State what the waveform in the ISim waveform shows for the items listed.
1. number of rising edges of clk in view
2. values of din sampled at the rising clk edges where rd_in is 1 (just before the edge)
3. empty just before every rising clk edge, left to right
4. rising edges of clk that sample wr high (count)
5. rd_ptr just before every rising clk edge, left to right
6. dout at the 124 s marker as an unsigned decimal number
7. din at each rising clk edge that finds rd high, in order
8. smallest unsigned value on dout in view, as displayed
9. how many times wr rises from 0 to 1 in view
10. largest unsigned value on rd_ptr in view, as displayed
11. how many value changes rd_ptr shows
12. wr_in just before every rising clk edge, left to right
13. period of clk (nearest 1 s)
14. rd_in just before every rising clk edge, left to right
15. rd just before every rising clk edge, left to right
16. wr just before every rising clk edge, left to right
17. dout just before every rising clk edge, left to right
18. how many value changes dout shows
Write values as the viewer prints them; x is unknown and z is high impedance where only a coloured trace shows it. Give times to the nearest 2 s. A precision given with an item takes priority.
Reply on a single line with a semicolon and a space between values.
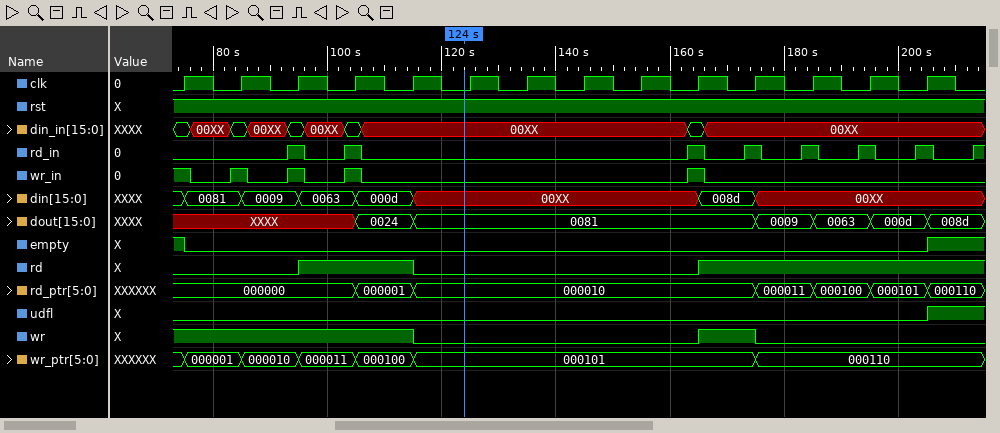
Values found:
14; 0009, 0063, 00XX, 008d, 00XX, 00XX, 00XX; 1 0 0 0 0 0 0 0 0 0 0 0 0 0; 6; 000000, 000000, 000000, 000000, 000001, 000010, 000010, 000010, 000010, 000010, 000010, 000011, 000100, 000101; 129; 0063, 000d, 008d, 00XX, 00XX, 00XX; 0009; 1; 000110; 6; 1 1 1 1 0 0 0 0 0 1 0 0 0 0; 10 s; 0 0 1 1 0 0 0 0 0 1 1 1 1 1; 0 0 0 1 1 0 0 0 0 0 1 1 1 1; 1 1 1 1 1 0 0 0 0 0 1 0 0 0; XXXX, XXXX, XXXX, XXXX, 0024, 0081, 0081, 0081, 0081, 0081, 0081, 0009, 0063, 000d; 6
